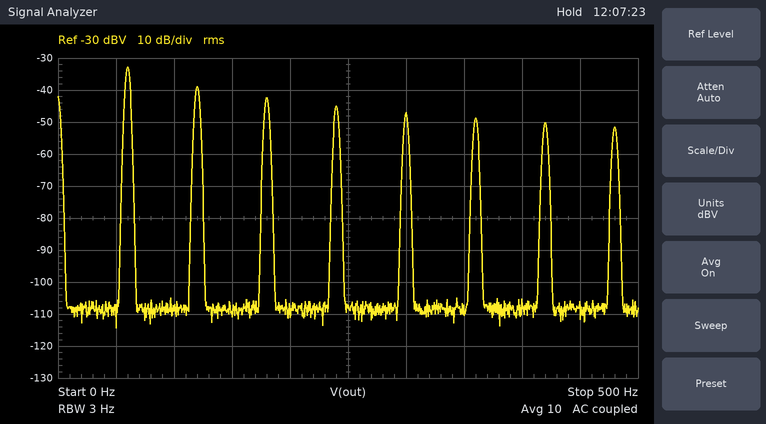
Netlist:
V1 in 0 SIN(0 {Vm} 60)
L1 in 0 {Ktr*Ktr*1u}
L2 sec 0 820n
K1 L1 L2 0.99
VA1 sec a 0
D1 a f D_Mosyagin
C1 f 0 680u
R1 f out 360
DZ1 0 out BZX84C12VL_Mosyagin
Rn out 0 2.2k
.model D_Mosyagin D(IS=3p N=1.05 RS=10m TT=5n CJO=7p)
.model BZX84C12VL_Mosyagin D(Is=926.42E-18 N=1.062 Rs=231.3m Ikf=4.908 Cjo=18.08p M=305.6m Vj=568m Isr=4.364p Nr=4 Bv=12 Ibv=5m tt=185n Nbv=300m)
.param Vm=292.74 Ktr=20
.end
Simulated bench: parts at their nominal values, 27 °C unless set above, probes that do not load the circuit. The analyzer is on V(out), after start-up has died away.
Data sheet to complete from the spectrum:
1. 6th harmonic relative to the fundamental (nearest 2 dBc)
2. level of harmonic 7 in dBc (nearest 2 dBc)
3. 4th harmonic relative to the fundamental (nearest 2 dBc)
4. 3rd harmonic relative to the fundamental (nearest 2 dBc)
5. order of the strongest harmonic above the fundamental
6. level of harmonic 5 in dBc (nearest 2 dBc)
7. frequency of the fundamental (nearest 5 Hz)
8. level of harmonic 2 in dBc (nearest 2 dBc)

-16 dBc
-18 dBc
-12 dBc
-10 dBc
2
-14 dBc
60 Hz
-6 dBc
